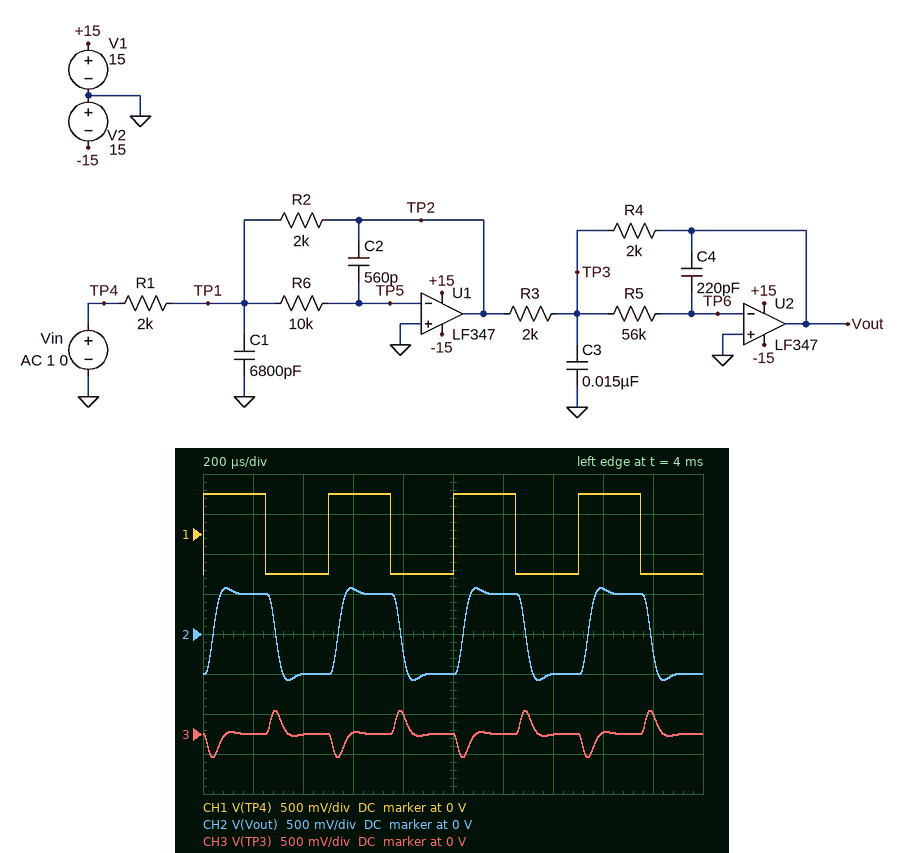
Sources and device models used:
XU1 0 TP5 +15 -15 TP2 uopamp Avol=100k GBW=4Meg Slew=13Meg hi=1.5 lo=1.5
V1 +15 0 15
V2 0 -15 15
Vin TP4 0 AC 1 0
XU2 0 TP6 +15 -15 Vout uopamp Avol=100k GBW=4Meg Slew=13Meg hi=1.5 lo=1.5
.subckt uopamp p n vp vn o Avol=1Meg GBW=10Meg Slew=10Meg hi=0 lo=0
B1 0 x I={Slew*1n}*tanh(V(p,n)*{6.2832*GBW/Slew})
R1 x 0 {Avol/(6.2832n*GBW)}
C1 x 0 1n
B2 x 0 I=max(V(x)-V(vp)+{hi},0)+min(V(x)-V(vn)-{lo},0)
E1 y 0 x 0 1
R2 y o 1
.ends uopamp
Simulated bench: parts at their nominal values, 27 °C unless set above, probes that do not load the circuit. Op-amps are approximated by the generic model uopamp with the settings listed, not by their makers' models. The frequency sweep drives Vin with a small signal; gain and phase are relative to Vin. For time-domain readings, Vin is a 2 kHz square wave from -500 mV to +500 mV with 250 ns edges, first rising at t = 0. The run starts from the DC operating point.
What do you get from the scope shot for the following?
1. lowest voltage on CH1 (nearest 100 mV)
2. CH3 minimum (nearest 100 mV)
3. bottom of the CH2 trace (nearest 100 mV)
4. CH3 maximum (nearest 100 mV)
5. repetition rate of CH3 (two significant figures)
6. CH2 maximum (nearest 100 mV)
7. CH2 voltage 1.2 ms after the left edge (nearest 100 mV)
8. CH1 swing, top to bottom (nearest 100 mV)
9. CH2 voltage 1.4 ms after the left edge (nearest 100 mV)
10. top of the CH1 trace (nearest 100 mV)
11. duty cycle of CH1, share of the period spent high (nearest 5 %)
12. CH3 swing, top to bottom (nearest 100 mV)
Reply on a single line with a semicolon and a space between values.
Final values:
-500 mV; -300 mV; -600 mV; 300 mV; 2.0 kHz; 600 mV; 500 mV; 1.0 V; -500 mV; 500 mV; 50 %; 600 mV
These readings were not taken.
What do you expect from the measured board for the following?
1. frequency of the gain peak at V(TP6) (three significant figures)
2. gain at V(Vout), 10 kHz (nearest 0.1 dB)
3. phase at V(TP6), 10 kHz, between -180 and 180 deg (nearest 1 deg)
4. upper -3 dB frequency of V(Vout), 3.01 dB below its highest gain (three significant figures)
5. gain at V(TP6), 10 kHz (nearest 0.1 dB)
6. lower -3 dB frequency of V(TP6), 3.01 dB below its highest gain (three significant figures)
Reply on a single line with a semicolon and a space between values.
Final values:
8.02 kHz; -4.7 dB; 115 deg; 8.63 kHz; -56.7 dB; 4.39 kHz
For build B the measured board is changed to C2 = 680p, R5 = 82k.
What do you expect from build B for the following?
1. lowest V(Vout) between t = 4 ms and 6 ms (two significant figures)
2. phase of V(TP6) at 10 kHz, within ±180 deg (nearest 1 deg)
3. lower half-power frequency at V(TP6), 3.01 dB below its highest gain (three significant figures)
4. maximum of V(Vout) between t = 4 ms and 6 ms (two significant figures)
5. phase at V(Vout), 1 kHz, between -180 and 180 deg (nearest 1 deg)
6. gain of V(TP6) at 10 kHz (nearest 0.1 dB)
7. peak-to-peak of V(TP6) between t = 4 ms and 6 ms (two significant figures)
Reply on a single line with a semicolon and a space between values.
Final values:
-520 mV; 97 deg; 3.18 kHz; 520 mV; -19 deg; -61.3 dB; 1.4 mV
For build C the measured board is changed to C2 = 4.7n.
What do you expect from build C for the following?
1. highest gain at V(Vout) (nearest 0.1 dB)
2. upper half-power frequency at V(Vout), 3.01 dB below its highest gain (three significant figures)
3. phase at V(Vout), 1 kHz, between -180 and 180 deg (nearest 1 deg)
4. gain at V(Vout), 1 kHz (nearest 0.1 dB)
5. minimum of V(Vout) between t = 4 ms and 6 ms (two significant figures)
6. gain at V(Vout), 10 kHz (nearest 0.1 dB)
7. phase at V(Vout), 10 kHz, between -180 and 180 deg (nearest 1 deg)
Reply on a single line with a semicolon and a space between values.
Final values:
0 dB; 1.65 kHz; -43 deg; -1.4 dB; -410 mV; -20.8 dB; 150 deg
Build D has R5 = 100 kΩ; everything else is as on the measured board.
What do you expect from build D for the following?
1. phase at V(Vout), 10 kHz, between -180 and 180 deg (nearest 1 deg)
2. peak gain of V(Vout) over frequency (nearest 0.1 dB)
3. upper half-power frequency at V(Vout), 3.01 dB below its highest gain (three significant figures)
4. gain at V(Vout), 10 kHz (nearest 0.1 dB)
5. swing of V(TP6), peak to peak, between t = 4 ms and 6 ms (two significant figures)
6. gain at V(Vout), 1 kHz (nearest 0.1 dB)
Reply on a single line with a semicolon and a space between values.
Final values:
-168 deg; 0 dB; 4.86 kHz; -10.5 dB; 1.2 mV; -0.1 dB
